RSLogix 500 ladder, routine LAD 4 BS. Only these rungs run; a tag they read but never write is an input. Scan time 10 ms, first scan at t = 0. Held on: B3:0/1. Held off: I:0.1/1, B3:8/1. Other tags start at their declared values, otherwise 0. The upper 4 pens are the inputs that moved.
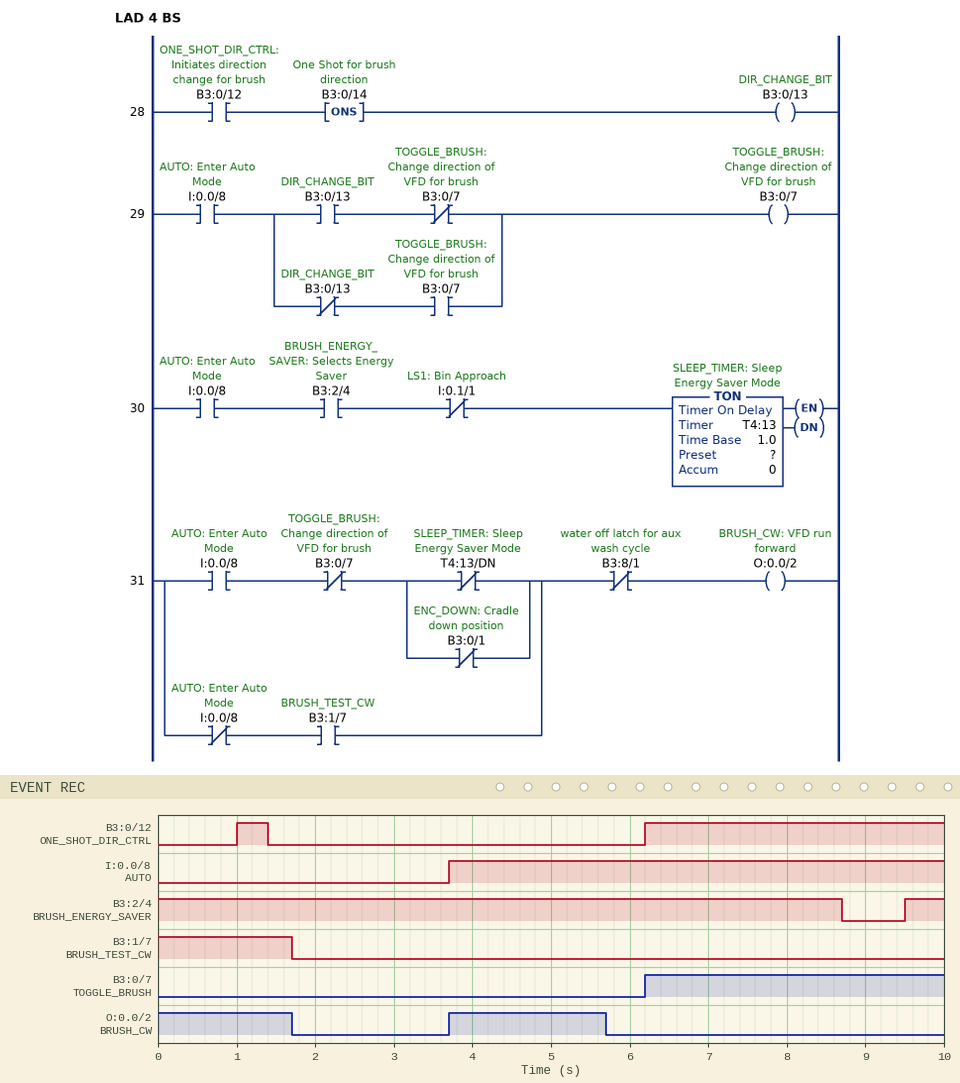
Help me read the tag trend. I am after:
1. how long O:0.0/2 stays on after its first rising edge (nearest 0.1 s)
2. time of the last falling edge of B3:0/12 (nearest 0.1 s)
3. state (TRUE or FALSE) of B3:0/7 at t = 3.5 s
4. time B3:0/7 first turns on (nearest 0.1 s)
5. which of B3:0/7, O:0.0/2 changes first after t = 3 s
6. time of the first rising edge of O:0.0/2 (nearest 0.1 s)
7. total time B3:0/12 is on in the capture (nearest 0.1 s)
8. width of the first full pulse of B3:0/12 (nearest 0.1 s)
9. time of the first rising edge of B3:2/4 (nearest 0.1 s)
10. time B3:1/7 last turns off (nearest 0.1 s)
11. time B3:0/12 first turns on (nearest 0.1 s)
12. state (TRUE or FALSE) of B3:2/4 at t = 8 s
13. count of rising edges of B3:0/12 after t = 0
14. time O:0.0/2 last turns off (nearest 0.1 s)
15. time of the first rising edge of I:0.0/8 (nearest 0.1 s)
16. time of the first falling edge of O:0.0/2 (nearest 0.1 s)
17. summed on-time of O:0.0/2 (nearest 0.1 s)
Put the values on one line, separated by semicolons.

2.0 s; 1.4 s; FALSE; 6.2 s; O:0.0/2; 3.7 s; 4.2 s; 0.4 s; 9.5 s; 1.7 s; 1.0 s; TRUE; 2; 5.7 s; 3.7 s; 1.7 s; 3.7 s
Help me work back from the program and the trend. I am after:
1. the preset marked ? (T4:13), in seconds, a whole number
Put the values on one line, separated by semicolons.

2 s
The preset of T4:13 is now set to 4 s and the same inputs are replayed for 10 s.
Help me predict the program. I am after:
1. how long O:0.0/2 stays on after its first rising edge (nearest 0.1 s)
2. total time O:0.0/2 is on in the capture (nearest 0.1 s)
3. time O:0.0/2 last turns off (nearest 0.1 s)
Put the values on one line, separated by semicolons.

2.5 s; 4.2 s; 6.2 s
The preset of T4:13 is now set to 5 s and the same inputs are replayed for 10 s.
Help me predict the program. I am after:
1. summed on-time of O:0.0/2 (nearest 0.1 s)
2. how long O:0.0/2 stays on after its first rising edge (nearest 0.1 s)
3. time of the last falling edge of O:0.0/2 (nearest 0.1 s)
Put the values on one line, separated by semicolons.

4.2 s; 2.5 s; 6.2 s
